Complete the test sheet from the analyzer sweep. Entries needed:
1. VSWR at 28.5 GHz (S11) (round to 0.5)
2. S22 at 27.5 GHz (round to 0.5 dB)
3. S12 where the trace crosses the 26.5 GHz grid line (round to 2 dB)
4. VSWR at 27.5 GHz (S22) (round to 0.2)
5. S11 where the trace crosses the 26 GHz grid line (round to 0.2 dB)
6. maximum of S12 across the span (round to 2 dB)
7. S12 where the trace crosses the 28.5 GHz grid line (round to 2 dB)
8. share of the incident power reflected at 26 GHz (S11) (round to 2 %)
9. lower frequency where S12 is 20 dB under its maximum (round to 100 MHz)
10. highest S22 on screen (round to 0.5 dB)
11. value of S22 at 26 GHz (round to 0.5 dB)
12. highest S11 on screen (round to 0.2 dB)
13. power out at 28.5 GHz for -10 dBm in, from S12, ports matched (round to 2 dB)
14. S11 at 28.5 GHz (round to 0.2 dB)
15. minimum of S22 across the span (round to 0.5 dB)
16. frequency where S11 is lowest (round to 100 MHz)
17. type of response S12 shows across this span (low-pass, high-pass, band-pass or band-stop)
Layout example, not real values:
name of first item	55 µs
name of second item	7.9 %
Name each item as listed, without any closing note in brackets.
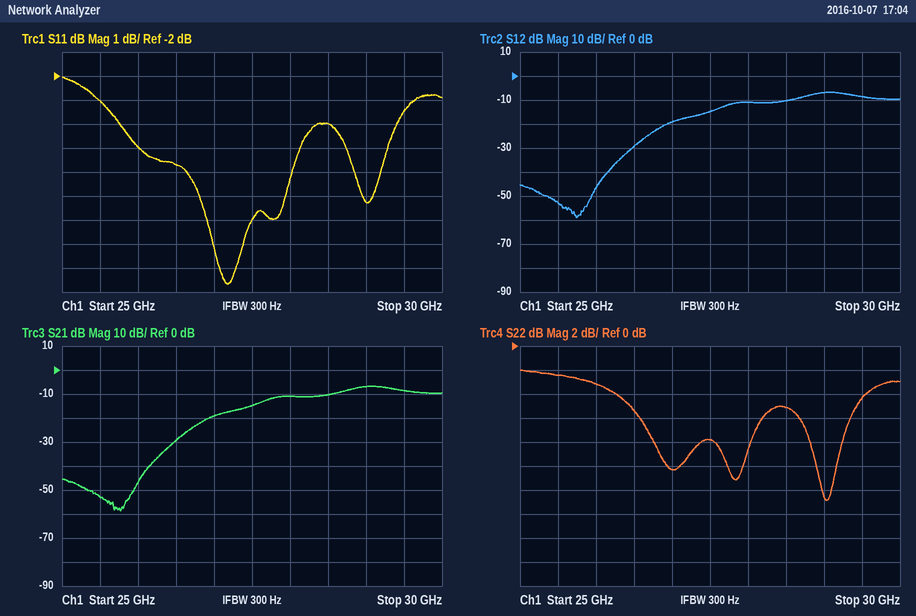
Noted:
VSWR at 28.5 GHz (S11)	4.5
S22 at 27.5 GHz	-8.0 dB
S12 where the trace crosses the 26.5 GHz grid line	-30 dB
VSWR at 27.5 GHz (S22)	2.4
S11 where the trace crosses the 26 GHz grid line	-5.0 dB
maximum of S12 across the span	-6 dB
S12 where the trace crosses the 28.5 GHz grid line	-10 dB
share of the incident power reflected at 26 GHz (S11)	32 %
lower frequency where S12 is 20 dB under its maximum	26.6 GHz
highest S22 on screen	-2.0 dB
value of S22 at 26 GHz	-3.0 dB
highest S11 on screen	-2.0 dB
power out at 28.5 GHz for -10 dBm in, from S12, ports matched	-20 dBm
S11 at 28.5 GHz	-4.0 dB
minimum of S22 across the span	-13.0 dB
frequency where S11 is lowest	27.2 GHz
type of response S12 shows across this span	high-pass
